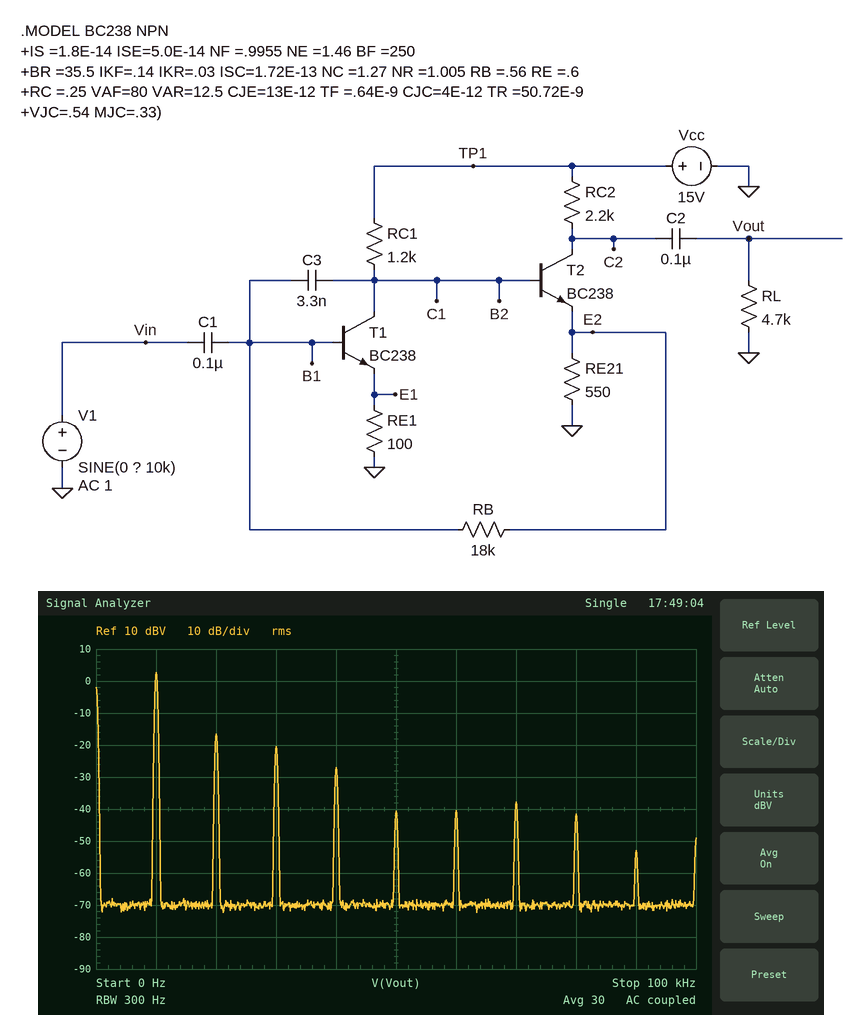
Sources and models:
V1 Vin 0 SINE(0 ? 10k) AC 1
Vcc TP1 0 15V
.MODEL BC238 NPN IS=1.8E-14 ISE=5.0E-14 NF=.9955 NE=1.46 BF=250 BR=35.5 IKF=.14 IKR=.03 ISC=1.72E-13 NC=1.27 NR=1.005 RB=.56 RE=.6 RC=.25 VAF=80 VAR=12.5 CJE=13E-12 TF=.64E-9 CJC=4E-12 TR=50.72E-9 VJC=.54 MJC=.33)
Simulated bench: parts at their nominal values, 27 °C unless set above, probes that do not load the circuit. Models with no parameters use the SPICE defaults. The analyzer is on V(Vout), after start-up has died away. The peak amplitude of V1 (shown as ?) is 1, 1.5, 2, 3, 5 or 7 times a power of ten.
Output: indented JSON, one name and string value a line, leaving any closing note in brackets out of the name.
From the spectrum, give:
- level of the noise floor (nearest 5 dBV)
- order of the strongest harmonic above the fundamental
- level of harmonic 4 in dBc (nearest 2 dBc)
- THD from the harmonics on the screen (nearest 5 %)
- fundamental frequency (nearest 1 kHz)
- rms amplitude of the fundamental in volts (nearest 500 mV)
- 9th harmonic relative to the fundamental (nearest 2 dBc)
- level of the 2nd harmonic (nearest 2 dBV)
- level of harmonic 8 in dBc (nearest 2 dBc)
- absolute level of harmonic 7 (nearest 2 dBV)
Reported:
{
  "level of the noise floor": "-70 dBV",
  "order of the strongest harmonic above the fundamental": "2",
  "level of harmonic 4 in dBc": "-30 dBc",
  "THD from the harmonics on the screen": "15 %",
  "fundamental frequency": "10 kHz",
  "rms amplitude of the fundamental in volts": "1.5 V",
  "9th harmonic relative to the fundamental": "-56 dBc",
  "level of the 2nd harmonic": "-16 dBV",
  "level of harmonic 8 in dBc": "-44 dBc",
  "absolute level of harmonic 7": "-38 dBV"
}
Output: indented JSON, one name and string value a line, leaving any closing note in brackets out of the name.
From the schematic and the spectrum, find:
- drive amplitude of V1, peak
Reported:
{
  "drive amplitude of V1, peak": "100 mV"
}
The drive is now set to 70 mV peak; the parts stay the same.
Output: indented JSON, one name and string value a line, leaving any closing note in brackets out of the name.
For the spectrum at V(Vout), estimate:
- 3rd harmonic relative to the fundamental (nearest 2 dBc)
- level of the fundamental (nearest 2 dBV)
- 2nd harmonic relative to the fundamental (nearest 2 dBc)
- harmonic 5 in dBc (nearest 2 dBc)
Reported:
{
  "3rd harmonic relative to the fundamental": "-44 dBc",
  "level of the fundamental": "0 dBV",
  "2nd harmonic relative to the fundamental": "-42 dBc",
  "harmonic 5 in dBc": "-46 dBc"
}
